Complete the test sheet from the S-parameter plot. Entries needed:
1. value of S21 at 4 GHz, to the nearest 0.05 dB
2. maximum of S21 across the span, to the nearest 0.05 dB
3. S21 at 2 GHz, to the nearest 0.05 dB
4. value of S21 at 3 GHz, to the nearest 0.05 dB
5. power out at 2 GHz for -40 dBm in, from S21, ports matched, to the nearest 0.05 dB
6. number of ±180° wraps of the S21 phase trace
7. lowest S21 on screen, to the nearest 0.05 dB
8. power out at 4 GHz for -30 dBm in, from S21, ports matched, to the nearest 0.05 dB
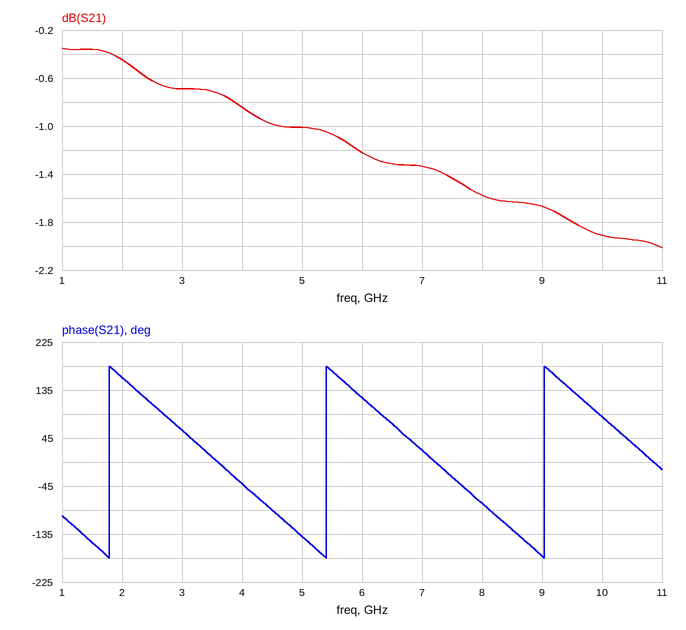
-0.85 dB
-0.35 dB
-0.45 dB
-0.70 dB
-40.45 dBm
3
-2.00 dB
-30.85 dBm
